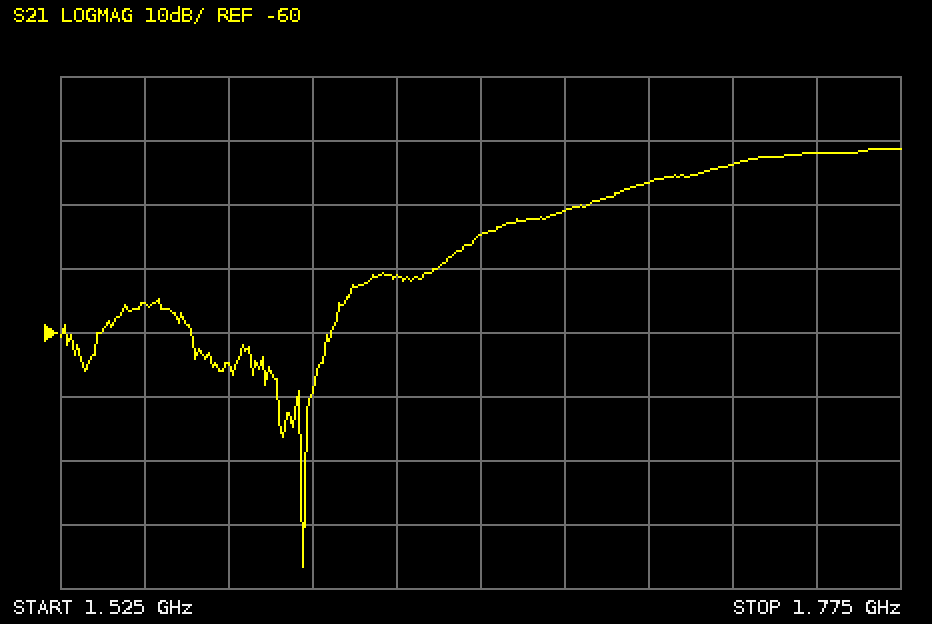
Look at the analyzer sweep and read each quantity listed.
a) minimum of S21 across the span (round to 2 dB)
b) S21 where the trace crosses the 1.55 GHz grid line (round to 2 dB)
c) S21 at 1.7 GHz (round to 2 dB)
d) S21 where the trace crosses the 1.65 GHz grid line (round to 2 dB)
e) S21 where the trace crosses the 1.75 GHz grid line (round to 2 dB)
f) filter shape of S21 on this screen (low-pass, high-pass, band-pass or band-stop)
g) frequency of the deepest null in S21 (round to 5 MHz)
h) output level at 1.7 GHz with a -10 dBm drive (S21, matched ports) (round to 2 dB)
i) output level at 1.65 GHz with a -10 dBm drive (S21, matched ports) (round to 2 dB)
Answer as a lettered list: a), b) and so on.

a) -96 dB
b) -56 dB
c) -36 dB
d) -44 dB
e) -32 dB
f) high-pass
g) 1.595 GHz
h) -46 dBm
i) -54 dBm
